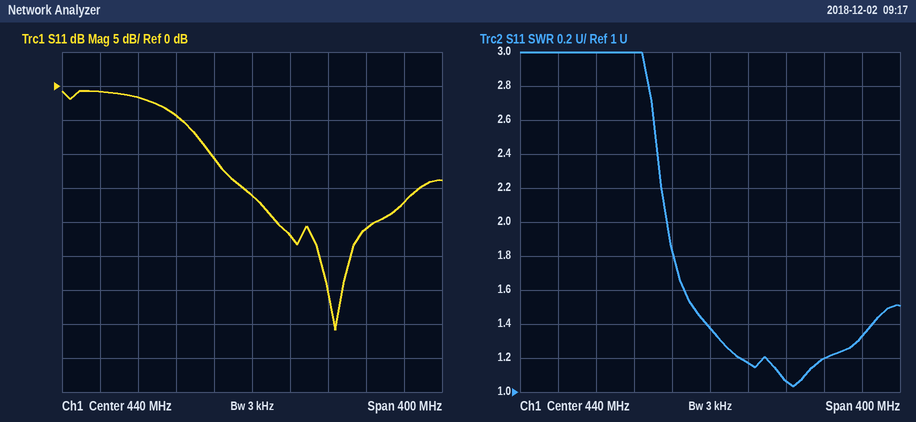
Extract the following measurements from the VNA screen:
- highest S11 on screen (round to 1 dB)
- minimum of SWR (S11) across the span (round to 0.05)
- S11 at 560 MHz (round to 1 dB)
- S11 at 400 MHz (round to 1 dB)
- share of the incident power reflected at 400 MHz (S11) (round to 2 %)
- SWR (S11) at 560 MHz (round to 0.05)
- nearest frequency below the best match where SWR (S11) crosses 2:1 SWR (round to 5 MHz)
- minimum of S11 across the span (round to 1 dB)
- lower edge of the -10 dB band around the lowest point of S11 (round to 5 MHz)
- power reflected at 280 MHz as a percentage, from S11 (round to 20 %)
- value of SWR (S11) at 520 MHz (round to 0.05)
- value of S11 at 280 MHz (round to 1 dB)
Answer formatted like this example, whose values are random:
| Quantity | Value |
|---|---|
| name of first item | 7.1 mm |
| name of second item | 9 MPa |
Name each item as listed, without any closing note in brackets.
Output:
| Quantity | Value |
|---|---|
| highest S11 on screen | -1 dB |
| minimum of SWR (S11) across the span | 1.05 |
| S11 at 560 MHz | -21 dB |
| S11 at 400 MHz | -11 dB |
| share of the incident power reflected at 400 MHz (S11) | 8 % |
| SWR (S11) at 560 MHz | 1.20 |
| nearest frequency below the best match where SWR (S11) crosses 2:1 SWR | 395 MHz |
| minimum of S11 across the span | -36 dB |
| lower edge of the -10 dB band around the lowest point of S11 | 395 MHz |
| power reflected at 280 MHz as a percentage, from S11 | 80 % |
| value of SWR (S11) at 520 MHz | 1.05 |
| value of S11 at 280 MHz | -1 dB |
